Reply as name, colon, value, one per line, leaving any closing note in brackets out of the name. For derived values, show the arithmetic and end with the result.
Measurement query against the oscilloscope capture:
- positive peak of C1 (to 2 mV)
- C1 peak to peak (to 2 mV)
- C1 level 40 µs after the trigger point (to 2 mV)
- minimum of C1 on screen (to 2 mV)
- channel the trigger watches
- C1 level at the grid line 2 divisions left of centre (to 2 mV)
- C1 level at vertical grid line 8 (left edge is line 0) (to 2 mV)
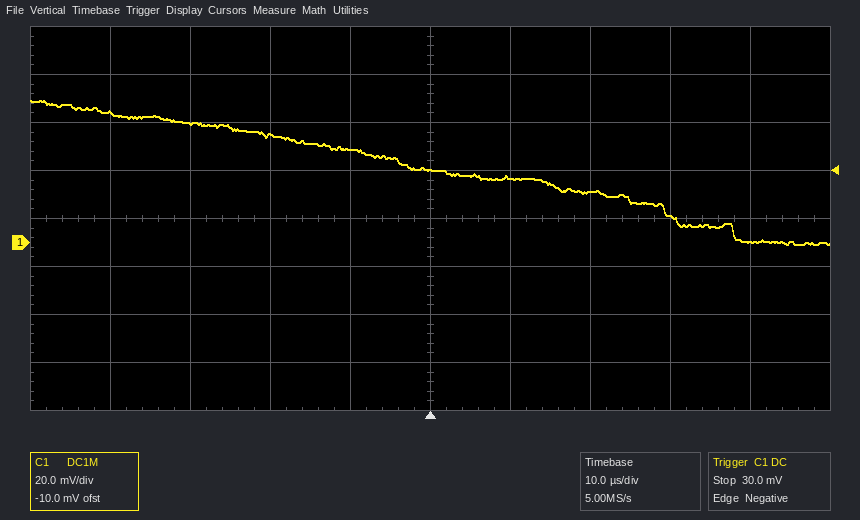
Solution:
positive peak of C1: 60 mV
C1 peak to peak: 60 mV − (0 mV) = 60 mV
C1 level 40 µs after the trigger point: 0 mV
minimum of C1 on screen: 0 mV
channel the trigger watches: C1
C1 level at the grid line 2 divisions left of centre: 44 mV
C1 level at vertical grid line 8 (left edge is line 0): 10 mV
